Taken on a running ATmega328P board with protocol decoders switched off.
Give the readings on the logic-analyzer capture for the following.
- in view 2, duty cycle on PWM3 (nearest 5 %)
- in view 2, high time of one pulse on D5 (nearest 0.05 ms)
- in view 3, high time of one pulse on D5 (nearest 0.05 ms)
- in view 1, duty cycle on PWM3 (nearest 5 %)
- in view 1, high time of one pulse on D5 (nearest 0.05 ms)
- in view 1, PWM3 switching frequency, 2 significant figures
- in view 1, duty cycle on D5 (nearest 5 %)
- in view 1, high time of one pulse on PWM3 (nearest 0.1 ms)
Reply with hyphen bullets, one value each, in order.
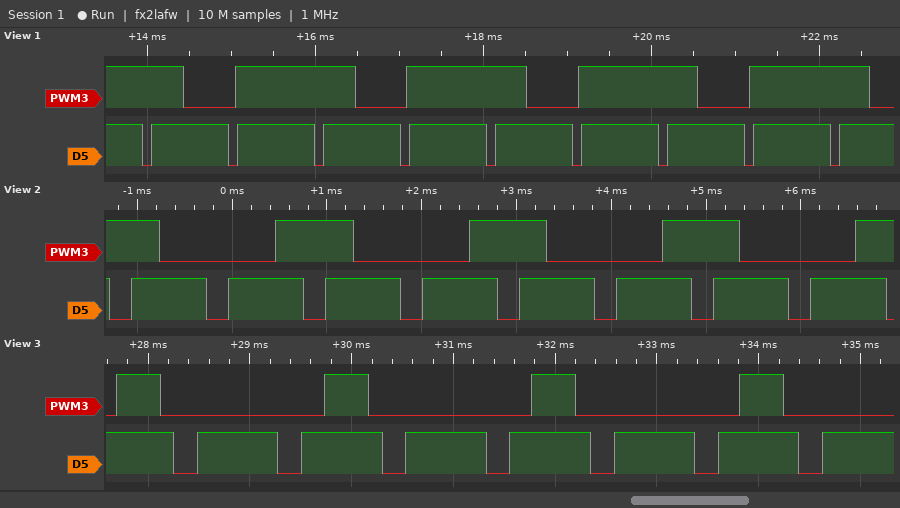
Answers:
- 40 %
- 0.80 ms
- 0.80 ms
- 70 %
- 0.90 ms
- 490 Hz
- 90 %
- 1.4 ms
